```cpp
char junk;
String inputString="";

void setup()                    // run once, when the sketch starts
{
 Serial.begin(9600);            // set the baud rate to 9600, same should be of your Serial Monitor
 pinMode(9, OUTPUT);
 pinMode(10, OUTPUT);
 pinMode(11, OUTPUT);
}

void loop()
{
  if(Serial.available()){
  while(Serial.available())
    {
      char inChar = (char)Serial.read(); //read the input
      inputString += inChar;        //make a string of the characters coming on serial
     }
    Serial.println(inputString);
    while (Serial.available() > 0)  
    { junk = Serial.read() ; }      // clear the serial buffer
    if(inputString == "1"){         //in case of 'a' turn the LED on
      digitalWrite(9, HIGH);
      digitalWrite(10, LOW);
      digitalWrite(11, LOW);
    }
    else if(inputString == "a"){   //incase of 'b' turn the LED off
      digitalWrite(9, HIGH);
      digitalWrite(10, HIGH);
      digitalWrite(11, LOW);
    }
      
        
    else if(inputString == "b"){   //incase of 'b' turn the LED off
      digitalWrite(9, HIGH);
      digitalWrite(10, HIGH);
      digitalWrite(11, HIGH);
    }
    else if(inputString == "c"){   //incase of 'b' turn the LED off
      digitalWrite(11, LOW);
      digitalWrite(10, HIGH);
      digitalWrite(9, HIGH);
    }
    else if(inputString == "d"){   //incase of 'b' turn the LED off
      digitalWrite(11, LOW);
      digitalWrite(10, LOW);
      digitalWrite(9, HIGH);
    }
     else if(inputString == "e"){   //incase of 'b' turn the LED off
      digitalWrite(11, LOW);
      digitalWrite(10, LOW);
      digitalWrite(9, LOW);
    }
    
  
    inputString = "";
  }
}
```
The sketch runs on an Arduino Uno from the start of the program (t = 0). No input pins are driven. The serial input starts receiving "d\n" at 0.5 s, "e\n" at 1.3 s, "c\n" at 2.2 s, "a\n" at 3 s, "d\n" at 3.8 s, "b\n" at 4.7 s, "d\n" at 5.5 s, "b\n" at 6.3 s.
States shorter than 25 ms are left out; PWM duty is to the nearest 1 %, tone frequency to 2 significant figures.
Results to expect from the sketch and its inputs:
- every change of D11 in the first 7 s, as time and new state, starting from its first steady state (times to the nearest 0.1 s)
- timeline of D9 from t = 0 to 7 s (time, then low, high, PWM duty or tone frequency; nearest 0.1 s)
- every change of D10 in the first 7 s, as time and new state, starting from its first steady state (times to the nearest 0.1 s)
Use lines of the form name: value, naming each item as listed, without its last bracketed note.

every change of D11 in the first 7 s, as time and new state, starting from its first steady state: 0 s low; 4.7 s high; 5.5 s low; 6.3 s high
timeline of D9 from t = 0 to 7 s: 0 s low; 0.5 s high; 1.3 s low; 2.2 s high
every change of D10 in the first 7 s, as time and new state, starting from its first steady state: 0 s low; 2.2 s high; 3.8 s low; 4.7 s high; 5.5 s low; 6.3 s high
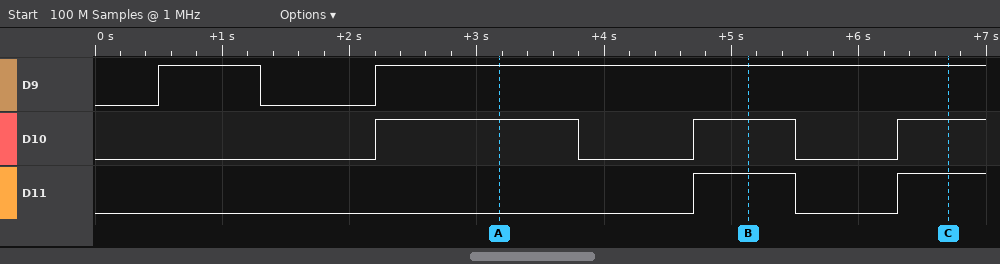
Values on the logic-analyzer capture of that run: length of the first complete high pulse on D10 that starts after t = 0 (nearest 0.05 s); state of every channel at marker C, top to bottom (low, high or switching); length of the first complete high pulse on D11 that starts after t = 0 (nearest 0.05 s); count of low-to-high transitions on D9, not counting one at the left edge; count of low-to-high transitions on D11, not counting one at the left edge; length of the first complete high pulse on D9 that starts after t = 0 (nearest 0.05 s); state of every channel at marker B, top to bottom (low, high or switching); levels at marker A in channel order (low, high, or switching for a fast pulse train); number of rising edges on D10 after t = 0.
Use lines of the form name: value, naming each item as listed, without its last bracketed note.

length of the first complete high pulse on D10 that starts after t = 0: 1.60 s
state of every channel at marker C, top to bottom: D9 high, D10 high, D11 high
length of the first complete high pulse on D11 that starts after t = 0: 0.80 s
count of low-to-high transitions on D9, not counting one at the left edge: 2
count of low-to-high transitions on D11, not counting one at the left edge: 2
length of the first complete high pulse on D9 that starts after t = 0: 0.80 s
state of every channel at marker B, top to bottom: D9 high, D10 high, D11 high
levels at marker A in channel order: D9 high, D10 high, D11 low
number of rising edges on D10 after t = 0: 3
